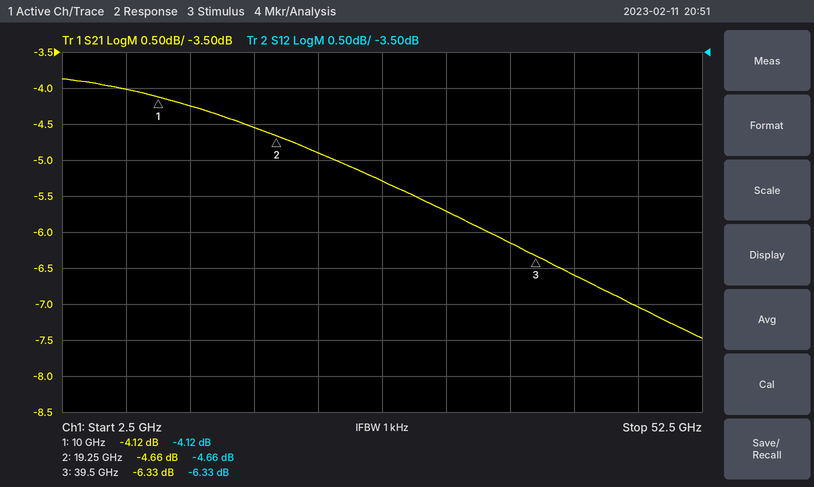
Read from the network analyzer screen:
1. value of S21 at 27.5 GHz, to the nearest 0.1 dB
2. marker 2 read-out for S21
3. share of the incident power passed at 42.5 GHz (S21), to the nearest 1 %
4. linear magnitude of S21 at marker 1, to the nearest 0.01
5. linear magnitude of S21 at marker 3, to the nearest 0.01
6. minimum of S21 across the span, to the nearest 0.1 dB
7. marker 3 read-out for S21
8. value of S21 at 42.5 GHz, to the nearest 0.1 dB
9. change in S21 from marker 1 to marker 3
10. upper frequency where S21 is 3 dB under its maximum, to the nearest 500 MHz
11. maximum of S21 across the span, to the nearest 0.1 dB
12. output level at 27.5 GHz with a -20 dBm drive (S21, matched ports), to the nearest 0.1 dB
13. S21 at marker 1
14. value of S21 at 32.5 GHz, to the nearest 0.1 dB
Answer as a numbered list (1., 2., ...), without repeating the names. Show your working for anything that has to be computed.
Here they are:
1. -5.3 dB
2. -4.66 dB
3. 10^(-6.6/10) ≈ 22 %
4. 10^(-4.12/20) ≈ 0.62
5. 10^(-6.33/20) ≈ 0.48
6. -7.5 dB
7. -6.33 dB
8. -6.6 dB
9. -6.33 − (-4.12) = -2.21 dB
10. 45.5 GHz
11. -3.9 dB
12. -20 dBm + (-5.3 dB) = -25.3 dBm
13. -4.12 dB
14. -5.7 dB
